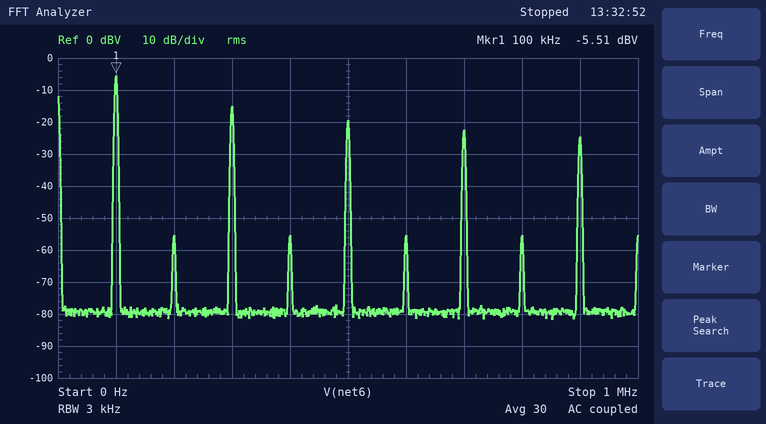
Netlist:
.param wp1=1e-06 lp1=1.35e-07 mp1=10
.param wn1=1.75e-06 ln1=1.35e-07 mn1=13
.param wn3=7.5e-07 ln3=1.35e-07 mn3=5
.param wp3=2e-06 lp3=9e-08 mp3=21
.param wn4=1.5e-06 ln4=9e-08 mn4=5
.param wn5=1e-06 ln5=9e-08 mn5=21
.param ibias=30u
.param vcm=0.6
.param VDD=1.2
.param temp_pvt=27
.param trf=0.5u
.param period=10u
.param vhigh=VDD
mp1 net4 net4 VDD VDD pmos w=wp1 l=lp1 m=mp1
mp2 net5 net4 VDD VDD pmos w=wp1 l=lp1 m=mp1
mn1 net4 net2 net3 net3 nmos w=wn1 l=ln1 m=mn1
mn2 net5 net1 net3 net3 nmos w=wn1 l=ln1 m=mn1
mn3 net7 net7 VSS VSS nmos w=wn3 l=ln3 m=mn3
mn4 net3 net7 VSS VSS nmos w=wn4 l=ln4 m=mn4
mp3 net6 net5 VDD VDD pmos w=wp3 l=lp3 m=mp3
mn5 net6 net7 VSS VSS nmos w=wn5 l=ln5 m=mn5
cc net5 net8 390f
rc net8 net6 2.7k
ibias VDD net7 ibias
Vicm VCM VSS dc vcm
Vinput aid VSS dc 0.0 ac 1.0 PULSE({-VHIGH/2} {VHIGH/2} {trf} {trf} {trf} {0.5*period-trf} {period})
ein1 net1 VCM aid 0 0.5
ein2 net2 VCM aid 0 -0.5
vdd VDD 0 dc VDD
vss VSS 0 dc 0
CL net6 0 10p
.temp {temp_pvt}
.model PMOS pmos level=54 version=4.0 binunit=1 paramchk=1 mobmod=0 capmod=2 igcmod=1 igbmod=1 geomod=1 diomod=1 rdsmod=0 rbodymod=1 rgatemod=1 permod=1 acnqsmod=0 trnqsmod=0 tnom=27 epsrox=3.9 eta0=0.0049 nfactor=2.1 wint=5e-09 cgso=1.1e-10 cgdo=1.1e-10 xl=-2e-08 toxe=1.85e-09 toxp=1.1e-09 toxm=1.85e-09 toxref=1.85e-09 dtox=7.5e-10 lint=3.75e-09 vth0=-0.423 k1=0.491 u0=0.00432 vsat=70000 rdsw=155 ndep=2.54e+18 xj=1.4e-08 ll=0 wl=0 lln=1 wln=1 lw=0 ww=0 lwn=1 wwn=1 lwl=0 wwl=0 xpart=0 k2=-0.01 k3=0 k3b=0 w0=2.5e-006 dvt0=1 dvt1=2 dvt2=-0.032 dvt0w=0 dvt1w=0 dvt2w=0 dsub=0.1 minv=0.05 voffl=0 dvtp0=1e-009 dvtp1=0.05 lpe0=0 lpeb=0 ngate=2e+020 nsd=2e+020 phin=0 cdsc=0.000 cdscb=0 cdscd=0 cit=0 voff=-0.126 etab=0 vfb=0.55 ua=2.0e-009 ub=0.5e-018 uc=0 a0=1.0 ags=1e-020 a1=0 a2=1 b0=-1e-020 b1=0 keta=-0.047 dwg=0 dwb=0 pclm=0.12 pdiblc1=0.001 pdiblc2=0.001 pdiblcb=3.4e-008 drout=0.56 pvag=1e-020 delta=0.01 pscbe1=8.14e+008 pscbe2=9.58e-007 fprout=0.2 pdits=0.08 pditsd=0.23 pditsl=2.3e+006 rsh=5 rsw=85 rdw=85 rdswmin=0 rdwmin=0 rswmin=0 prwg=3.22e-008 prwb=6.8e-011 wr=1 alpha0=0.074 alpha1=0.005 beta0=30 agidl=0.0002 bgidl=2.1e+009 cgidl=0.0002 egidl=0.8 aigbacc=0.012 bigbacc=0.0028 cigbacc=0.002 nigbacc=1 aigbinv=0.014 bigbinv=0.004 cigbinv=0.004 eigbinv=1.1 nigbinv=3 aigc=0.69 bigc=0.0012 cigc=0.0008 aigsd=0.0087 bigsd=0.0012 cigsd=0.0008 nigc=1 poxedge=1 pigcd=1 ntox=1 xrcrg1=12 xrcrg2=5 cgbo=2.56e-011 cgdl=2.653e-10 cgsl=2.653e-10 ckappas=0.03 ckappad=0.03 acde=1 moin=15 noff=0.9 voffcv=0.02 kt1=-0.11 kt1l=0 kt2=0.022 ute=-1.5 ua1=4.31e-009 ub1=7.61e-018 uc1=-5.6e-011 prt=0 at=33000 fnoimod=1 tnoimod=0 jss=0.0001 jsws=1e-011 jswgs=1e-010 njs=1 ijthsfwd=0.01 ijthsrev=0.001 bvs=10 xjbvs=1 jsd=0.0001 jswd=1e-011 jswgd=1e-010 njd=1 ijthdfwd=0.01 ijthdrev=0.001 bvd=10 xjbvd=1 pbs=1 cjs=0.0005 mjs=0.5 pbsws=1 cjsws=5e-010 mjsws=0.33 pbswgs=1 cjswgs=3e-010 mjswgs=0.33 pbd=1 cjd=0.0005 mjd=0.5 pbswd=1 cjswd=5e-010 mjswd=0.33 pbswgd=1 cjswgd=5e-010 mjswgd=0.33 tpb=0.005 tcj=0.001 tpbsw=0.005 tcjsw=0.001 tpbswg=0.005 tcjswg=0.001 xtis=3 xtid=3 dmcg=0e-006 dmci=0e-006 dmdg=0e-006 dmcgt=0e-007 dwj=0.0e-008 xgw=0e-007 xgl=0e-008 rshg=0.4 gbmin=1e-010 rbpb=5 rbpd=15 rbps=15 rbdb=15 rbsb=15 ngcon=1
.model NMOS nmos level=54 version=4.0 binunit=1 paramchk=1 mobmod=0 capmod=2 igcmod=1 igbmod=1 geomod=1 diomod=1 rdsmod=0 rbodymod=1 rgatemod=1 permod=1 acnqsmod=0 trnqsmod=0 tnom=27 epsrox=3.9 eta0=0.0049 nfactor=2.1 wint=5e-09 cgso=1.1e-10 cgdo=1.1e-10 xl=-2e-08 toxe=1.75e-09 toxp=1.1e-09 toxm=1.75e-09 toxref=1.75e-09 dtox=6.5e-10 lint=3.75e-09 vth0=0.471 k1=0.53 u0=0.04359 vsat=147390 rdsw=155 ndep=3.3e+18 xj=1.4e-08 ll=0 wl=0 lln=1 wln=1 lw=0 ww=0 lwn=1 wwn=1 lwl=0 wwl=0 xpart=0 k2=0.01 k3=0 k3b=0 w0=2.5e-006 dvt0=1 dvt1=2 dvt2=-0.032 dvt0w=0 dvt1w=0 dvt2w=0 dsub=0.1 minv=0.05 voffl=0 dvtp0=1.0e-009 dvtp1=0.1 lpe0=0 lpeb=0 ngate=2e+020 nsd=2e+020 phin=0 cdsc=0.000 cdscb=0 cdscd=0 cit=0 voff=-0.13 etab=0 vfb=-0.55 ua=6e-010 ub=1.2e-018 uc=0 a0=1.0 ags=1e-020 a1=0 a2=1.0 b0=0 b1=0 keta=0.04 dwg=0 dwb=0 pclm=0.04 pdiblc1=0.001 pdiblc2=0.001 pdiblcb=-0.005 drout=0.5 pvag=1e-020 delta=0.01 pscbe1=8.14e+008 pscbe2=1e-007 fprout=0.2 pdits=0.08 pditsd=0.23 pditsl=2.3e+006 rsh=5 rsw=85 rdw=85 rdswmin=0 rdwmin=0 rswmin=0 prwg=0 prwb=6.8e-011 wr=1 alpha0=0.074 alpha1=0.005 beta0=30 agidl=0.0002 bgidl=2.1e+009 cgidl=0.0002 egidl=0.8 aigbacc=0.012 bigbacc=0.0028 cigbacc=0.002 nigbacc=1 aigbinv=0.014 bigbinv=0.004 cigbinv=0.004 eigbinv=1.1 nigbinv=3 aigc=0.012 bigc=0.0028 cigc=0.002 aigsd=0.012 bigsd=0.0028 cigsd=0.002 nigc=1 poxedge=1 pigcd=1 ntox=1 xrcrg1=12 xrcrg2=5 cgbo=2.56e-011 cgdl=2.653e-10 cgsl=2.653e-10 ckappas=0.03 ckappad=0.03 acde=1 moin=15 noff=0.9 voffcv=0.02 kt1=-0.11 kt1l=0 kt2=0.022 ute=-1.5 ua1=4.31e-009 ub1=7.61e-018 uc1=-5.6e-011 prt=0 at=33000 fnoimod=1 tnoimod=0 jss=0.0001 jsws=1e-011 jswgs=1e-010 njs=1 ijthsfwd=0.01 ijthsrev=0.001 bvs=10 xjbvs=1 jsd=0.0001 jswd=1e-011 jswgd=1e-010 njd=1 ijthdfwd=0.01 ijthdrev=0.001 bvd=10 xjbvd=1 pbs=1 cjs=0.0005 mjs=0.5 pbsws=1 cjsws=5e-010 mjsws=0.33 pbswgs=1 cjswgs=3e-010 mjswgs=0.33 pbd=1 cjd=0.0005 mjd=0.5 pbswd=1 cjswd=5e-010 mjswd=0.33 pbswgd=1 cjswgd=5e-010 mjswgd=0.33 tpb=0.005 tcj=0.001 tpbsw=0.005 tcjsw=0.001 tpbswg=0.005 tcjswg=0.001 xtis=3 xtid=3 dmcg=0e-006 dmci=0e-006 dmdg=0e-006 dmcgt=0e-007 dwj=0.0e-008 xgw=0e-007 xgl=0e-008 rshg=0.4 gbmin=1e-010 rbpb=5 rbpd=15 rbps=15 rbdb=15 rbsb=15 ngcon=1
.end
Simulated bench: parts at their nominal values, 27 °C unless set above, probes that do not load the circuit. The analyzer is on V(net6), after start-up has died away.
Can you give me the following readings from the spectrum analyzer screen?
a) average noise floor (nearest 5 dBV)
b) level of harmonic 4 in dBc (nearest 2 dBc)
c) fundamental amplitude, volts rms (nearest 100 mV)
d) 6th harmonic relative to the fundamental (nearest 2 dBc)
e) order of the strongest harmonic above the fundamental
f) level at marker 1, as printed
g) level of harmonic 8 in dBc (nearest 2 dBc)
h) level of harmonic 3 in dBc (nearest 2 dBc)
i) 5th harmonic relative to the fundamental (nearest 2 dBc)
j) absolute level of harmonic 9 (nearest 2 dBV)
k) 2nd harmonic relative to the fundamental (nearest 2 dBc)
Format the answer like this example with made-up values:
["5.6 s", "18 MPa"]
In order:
["-80 dBV", "-50 dBc", "500 mV", "-50 dBc", "3", "-5.51 dBV", "-50 dBc", "-10 dBc", "-14 dBc", "-24 dBV", "-50 dBc"]
